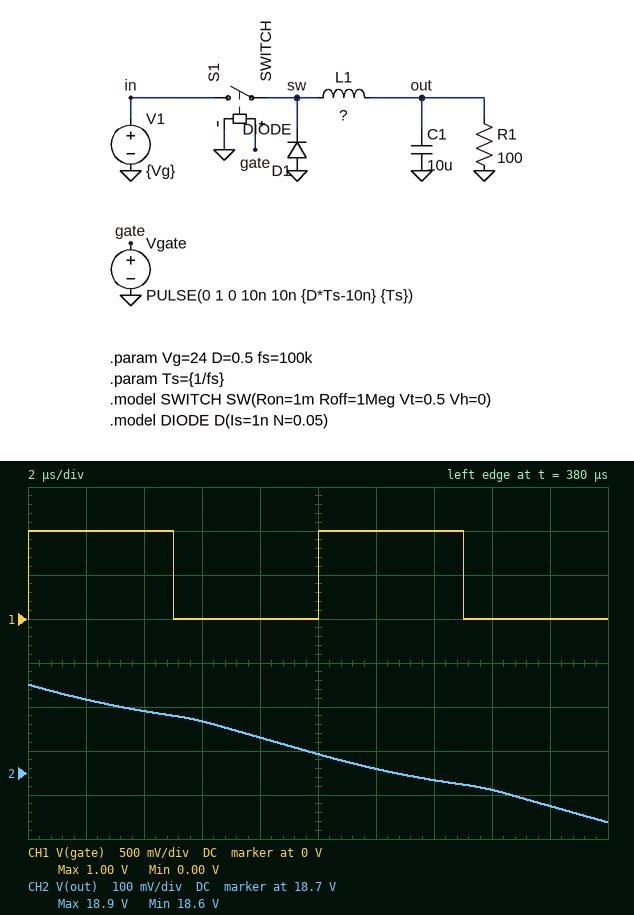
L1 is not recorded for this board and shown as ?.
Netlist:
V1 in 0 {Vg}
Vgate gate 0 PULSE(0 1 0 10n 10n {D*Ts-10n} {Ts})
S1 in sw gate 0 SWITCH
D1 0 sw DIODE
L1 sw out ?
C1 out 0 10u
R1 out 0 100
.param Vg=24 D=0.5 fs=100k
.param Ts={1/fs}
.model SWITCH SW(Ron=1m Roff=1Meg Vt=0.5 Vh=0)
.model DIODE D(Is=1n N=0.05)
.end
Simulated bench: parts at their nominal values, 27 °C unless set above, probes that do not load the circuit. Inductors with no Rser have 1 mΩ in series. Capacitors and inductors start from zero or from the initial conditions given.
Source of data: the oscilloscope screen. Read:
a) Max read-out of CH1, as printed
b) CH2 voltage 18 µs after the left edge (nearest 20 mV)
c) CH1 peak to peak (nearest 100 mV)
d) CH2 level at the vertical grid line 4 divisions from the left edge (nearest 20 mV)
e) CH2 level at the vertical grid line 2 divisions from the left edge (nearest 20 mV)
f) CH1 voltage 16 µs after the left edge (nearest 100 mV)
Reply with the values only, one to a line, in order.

1.00 V
18.62 V
1.0 V
18.78 V
18.84 V
0 V
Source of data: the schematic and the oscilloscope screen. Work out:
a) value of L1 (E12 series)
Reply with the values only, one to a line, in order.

270 µH
